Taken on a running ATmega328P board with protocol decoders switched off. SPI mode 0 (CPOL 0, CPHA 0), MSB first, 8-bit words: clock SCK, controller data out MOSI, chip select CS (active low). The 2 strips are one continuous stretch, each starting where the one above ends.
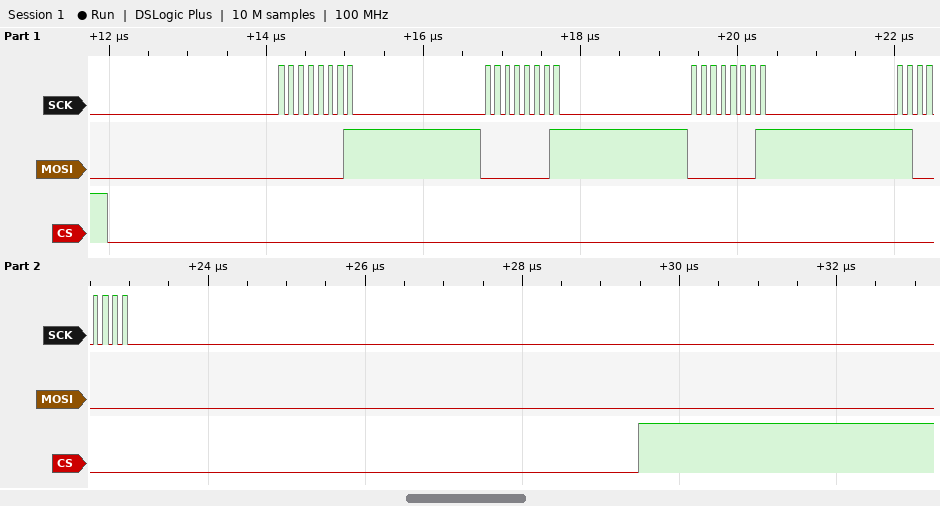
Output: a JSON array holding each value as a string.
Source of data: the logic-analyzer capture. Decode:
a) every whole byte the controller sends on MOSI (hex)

["01 01 01 C0"]
